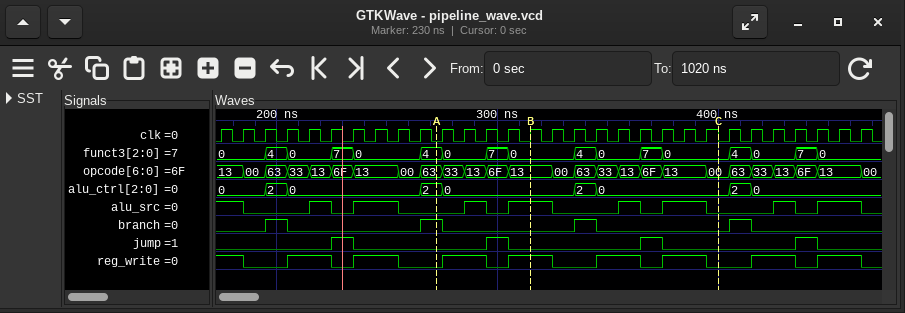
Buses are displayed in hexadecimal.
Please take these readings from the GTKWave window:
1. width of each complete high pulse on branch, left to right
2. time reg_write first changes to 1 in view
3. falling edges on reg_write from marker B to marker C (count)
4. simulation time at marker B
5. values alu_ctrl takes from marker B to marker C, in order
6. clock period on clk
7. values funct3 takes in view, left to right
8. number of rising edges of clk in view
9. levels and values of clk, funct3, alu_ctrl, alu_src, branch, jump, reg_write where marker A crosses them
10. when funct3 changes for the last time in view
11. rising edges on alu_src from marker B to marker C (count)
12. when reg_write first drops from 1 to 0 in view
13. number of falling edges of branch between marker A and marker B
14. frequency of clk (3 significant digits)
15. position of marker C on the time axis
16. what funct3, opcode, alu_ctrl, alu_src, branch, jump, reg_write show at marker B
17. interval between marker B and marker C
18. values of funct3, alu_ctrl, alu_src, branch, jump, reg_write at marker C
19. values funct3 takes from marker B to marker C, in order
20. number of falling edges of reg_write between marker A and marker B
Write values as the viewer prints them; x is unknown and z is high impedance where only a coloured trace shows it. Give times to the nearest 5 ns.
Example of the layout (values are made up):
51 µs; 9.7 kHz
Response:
10 ns, 10 ns, 10 ns, 10 ns; 205 ns; 3; 315 ns; 0, 2, 0; 10 ns; 0, 4, 0, 7, 0, 4, 0, 7, 0, 4, 0, 7, 0, 4, 0, 7, 0; 30; clk=0, funct3=4, alu_ctrl=2, alu_src=0, branch=1, jump=0, reg_write=0; 445 ns; 2; 185 ns; 1; 100 MHz; 400 ns; funct3=0, opcode=13, alu_ctrl=0, alu_src=1, branch=0, jump=0, reg_write=1; 85 ns; funct3=0, alu_ctrl=0, alu_src=0, branch=0, jump=0, reg_write=0; 0, 4, 0, 7, 0; 1
